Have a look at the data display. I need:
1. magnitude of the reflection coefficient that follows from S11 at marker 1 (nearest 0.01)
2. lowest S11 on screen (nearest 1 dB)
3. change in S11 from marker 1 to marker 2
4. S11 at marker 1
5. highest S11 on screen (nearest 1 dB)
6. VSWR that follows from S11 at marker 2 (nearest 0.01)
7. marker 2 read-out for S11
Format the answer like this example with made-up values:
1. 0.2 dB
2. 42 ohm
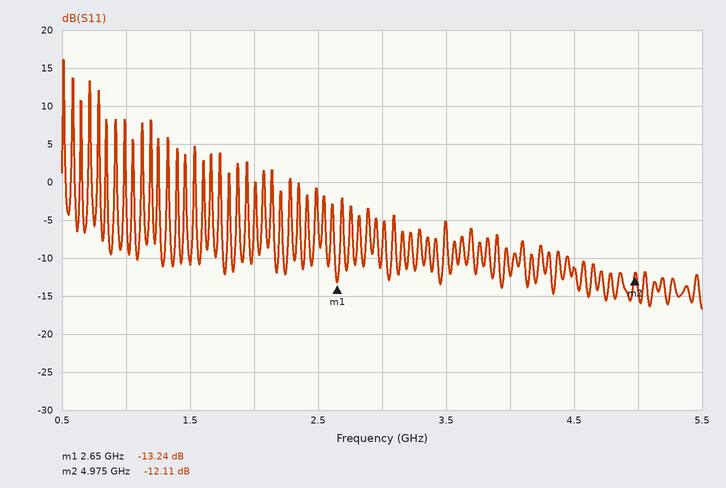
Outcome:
1. 0.22
2. -17 dB
3. 1.13 dB
4. -13.24 dB
5. 16 dB
6. 1.66
7. -12.11 dB
